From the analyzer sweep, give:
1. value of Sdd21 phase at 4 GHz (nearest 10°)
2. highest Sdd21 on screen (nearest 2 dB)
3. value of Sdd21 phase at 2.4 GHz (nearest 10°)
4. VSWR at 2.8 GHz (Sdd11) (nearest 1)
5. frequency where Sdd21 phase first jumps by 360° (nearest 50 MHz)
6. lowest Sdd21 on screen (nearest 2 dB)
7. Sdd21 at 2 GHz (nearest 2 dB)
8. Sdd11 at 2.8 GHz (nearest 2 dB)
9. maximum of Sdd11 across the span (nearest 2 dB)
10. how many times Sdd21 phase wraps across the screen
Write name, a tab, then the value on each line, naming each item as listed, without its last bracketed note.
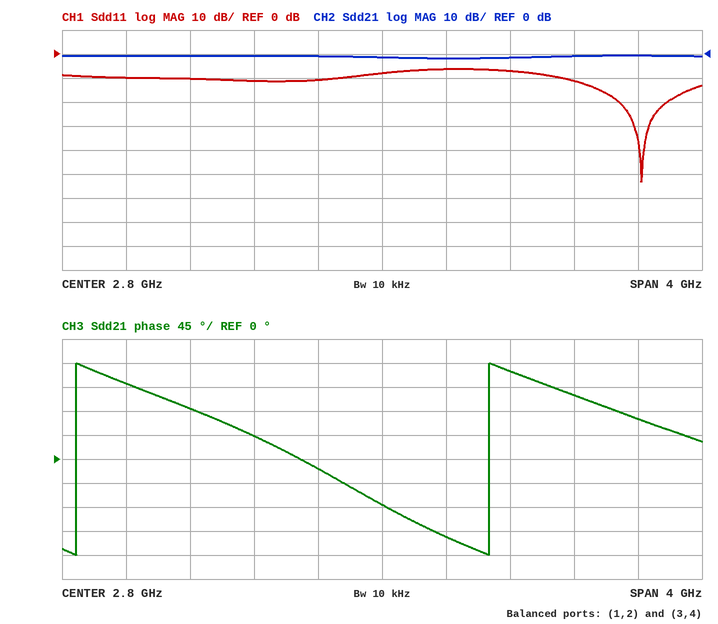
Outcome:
value of Sdd21 phase at 4 GHz	120°
highest Sdd21 on screen	0 dB
value of Sdd21 phase at 2.4 GHz	-20°
VSWR at 2.8 GHz (Sdd11)	2
frequency where Sdd21 phase first jumps by 360°	900 MHz
lowest Sdd21 on screen	-2 dB
Sdd21 at 2 GHz	0 dB
Sdd11 at 2.8 GHz	-8 dB
maximum of Sdd11 across the span	-6 dB
how many times Sdd21 phase wraps across the screen	2
